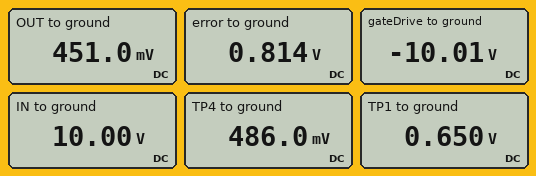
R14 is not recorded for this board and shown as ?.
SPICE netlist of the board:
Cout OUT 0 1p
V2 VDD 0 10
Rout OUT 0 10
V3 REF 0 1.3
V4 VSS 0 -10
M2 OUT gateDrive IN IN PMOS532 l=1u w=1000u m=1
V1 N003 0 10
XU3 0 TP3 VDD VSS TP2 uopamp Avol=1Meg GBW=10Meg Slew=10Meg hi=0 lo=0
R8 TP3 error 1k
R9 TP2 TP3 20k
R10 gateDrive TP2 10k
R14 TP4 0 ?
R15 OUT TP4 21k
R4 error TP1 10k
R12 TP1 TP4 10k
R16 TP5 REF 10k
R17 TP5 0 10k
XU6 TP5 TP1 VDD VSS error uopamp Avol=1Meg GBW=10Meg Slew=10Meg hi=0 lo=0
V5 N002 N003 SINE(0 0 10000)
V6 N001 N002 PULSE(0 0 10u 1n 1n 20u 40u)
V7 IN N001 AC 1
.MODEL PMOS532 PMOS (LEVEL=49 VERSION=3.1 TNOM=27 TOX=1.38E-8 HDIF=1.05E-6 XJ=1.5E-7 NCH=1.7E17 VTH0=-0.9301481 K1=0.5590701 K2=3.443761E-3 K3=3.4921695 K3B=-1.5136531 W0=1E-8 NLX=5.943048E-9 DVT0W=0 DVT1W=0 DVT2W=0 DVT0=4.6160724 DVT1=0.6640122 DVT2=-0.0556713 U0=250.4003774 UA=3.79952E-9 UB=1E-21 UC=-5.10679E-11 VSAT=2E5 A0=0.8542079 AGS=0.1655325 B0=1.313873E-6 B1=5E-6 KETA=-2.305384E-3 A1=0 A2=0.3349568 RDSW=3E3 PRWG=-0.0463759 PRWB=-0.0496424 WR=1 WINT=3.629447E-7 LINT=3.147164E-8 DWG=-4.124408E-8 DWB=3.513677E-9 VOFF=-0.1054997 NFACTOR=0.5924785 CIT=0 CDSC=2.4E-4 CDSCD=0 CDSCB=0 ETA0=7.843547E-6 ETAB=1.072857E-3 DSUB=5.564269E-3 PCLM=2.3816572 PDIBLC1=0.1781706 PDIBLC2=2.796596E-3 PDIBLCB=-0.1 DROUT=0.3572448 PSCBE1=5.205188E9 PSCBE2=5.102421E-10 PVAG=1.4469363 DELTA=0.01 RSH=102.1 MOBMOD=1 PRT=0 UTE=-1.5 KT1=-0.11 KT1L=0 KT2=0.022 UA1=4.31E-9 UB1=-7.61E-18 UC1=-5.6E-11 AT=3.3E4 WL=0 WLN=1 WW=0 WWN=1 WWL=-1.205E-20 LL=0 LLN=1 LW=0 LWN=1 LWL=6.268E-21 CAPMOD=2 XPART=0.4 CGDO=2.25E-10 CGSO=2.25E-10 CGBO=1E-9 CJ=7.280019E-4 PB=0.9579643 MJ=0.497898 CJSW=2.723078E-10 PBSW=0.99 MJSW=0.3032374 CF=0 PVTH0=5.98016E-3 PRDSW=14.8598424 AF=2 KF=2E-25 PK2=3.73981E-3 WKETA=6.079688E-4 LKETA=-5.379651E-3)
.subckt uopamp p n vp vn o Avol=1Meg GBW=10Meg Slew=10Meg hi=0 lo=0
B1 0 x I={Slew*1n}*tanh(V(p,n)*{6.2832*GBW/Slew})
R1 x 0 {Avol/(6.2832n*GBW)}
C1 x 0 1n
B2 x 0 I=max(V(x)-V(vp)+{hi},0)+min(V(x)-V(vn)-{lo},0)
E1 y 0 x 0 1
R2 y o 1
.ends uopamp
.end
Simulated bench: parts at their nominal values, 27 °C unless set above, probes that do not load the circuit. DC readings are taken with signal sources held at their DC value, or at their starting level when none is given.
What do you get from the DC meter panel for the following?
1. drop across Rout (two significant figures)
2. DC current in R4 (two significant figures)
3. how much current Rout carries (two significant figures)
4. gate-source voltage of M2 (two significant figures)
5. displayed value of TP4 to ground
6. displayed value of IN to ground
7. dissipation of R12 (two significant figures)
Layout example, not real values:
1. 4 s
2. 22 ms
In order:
1. 450 mV
2. 16 µA
3. 45 mA
4. -20 V
5. 486.0 mV
6. 10.00 V
7. 2.7 µW
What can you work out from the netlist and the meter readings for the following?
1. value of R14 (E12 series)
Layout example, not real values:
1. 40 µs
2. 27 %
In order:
1. 33 kΩ
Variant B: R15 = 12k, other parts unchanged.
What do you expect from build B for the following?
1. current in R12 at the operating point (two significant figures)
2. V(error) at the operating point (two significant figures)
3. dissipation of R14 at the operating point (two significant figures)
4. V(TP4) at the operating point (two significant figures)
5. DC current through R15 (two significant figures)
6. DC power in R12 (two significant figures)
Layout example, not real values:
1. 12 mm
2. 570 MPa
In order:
1. 17 µA
2. 820 mV
3. 7.0 µW
4. 480 mV
5. 2.4 µA
6. 2.9 µW
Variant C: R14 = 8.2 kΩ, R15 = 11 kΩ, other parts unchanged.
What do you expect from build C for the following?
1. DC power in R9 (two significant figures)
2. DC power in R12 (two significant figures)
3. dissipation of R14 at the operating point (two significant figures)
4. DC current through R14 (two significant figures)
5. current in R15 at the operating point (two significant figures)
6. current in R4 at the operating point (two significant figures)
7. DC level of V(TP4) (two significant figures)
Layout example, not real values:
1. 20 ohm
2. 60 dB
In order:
1. 5.5 mW
2. 9.7 µW
3. 14 µW
4. 41 µA
5. 10 µA
6. 31 µA
7. 340 mV
